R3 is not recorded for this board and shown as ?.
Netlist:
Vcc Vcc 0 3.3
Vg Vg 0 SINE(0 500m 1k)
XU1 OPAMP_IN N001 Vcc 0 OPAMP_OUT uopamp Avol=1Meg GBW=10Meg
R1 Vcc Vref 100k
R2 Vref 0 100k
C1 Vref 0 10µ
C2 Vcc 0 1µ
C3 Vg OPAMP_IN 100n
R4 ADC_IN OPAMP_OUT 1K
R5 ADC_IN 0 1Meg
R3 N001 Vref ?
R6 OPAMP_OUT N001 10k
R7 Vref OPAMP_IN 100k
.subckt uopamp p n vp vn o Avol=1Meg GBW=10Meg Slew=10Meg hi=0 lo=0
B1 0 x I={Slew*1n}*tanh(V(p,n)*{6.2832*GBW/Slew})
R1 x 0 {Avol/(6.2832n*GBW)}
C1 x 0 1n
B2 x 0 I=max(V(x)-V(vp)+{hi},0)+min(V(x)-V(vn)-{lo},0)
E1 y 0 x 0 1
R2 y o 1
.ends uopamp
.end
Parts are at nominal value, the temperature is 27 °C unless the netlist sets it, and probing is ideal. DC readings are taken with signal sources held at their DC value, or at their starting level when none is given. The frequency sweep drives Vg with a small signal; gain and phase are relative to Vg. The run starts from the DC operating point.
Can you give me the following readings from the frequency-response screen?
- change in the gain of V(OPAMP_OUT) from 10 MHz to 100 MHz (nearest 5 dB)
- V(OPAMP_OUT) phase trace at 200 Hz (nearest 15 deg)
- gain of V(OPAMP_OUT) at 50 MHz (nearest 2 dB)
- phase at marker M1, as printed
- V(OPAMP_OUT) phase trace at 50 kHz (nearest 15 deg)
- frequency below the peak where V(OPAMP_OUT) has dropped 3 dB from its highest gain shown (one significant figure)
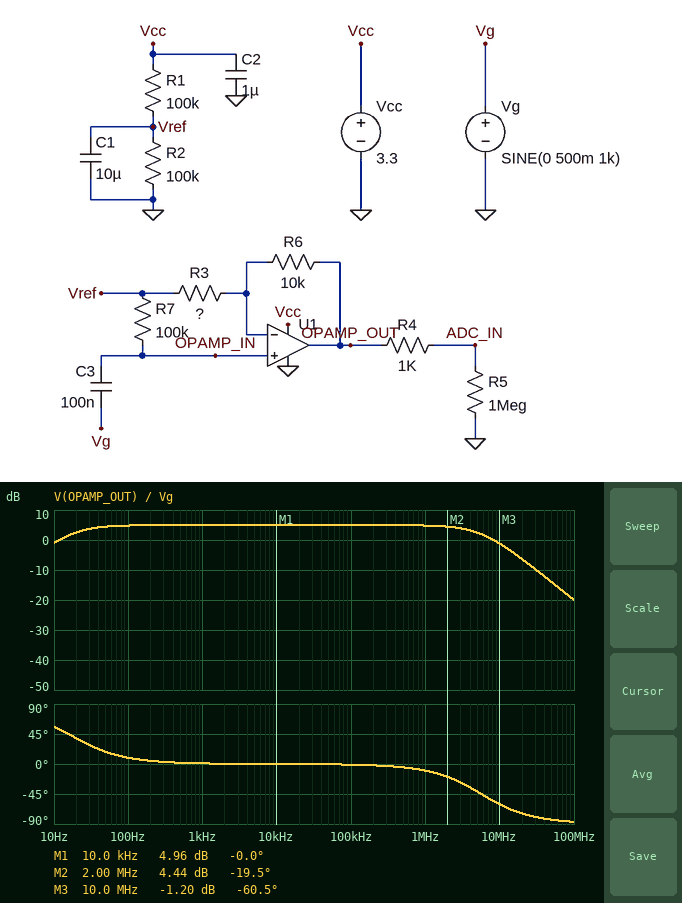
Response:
-20 dB
0 deg
-14 dB
-0.0 deg
0 deg
20 Hz
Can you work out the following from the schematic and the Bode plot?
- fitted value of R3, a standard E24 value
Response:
13 kΩ
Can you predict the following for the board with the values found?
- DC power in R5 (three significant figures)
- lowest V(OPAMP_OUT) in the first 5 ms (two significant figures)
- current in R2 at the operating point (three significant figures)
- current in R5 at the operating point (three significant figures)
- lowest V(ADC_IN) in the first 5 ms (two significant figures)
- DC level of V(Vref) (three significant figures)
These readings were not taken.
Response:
2.72 µW
750 mV
16.5 µA
1.65 µA
750 mV
1.65 V
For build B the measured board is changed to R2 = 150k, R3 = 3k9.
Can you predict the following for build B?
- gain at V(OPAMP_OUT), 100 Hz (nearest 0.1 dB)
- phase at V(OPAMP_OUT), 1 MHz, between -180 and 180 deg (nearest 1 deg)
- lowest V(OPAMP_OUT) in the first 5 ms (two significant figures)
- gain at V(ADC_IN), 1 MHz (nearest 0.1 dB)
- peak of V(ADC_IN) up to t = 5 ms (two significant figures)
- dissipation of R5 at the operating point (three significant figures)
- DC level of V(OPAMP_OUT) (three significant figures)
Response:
10.9 dB
-20 deg
170 mV
10.5 dB
3.3 V
3.91 µW
1.98 V
